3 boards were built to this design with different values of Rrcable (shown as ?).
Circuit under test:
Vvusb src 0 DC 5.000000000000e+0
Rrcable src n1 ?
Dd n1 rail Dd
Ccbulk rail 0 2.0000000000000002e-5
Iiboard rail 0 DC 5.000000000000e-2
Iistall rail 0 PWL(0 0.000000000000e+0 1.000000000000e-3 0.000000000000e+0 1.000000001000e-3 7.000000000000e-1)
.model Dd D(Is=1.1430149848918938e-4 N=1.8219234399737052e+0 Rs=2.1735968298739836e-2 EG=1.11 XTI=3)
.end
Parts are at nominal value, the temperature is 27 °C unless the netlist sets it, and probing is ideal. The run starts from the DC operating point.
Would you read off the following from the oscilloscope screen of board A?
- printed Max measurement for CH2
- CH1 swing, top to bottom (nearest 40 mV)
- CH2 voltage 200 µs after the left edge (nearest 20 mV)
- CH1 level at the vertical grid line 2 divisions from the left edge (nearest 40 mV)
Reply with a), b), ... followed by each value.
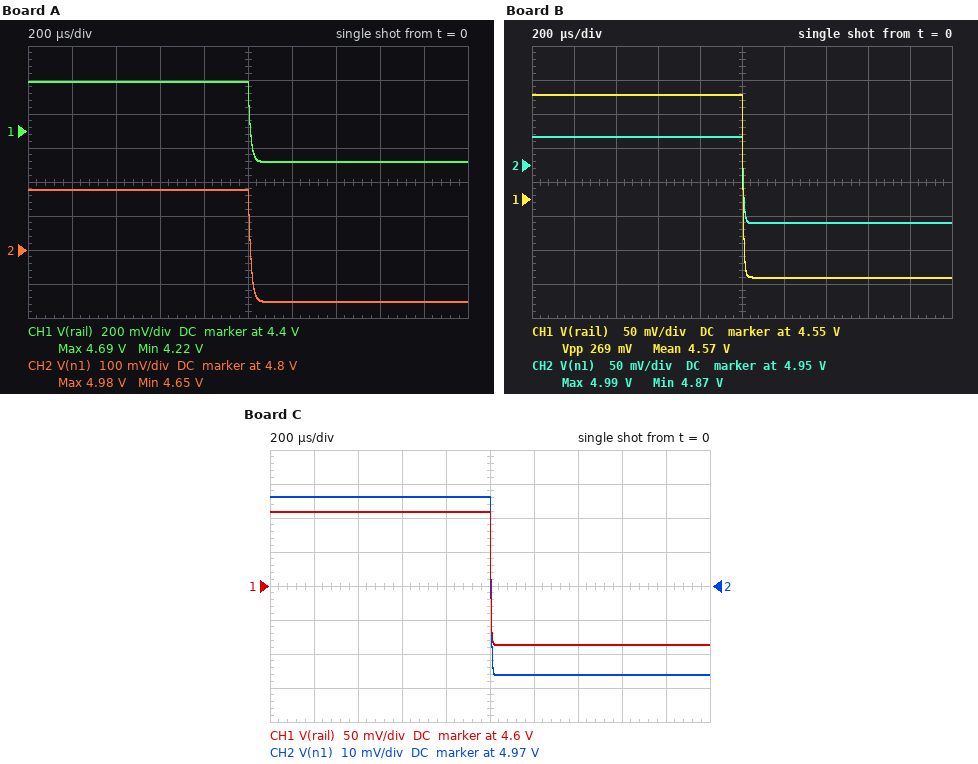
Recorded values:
a) 4.98 V
b) 480 mV
c) 4.98 V
d) 4.68 V
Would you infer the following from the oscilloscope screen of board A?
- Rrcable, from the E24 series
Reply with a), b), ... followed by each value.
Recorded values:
a) 0.47 Ω
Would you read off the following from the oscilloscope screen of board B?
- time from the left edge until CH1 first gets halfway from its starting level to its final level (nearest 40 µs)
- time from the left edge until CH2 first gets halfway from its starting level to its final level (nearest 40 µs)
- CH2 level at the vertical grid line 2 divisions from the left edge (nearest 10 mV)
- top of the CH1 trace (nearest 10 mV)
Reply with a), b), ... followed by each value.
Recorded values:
a) 1.00 ms
b) 1.00 ms
c) 4.99 V
d) 4.70 V
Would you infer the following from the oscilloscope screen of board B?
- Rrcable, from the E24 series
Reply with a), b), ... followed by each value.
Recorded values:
a) 0.18 Ω
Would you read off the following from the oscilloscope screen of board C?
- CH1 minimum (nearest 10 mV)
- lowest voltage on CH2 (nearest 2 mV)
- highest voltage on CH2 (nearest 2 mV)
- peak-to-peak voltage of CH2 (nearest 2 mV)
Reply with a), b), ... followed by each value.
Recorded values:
a) 4.51 V
b) 4.944 V
c) 4.996 V
d) 52 mV
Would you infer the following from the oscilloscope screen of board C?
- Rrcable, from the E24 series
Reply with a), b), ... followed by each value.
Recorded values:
a) 0.075 Ω
